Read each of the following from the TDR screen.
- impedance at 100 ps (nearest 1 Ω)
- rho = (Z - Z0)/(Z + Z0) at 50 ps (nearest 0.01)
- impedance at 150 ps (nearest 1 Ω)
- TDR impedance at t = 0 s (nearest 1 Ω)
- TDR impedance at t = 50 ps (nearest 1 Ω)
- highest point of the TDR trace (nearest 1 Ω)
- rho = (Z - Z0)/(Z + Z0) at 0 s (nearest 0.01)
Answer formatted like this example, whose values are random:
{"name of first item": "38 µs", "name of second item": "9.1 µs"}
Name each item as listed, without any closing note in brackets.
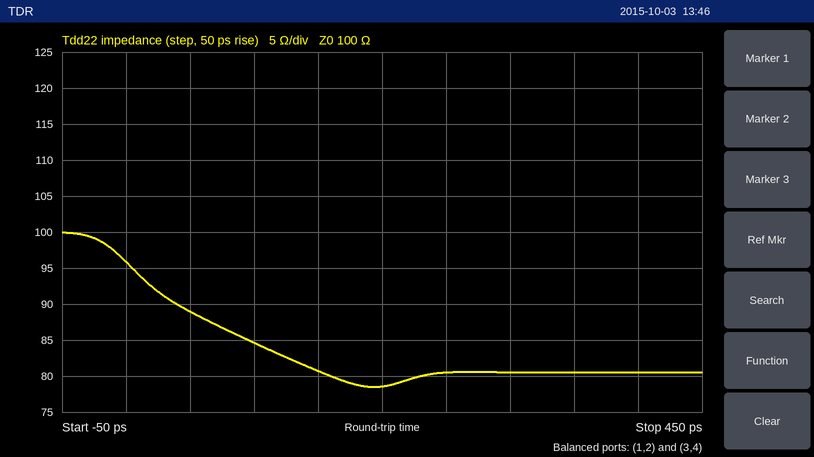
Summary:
{"impedance at 100 ps": "85 Ω", "rho = (Z - Z0)/(Z + Z0) at 50 ps": "-0.06", "impedance at 150 ps": "81 Ω", "TDR impedance at t = 0 s": "96 Ω", "TDR impedance at t = 50 ps": "89 Ω", "highest point of the TDR trace": "100 Ω", "rho = (Z - Z0)/(Z + Z0) at 0 s": "-0.02"}
